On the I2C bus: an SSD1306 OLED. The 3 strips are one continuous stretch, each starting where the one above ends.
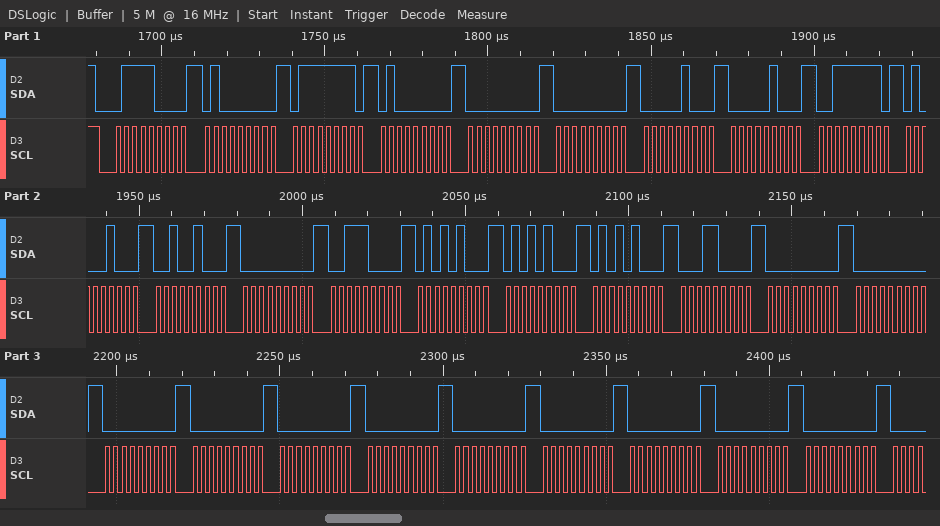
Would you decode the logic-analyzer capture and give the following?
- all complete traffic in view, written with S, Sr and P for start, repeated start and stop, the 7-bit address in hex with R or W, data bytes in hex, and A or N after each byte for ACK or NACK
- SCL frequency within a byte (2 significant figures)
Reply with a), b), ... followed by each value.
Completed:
a) S 3CW A 40 A 7F A 40 A 00 A 00 A 04 A 04 A 3F A 44 A 24 A 00 A 38 A 54 A 54 A 54 A 18 A 00 A 00 A 00 A 00 A 00 A 00 A 00 A 00 A 00 A 00 A 00 A
b) 400 kHz
